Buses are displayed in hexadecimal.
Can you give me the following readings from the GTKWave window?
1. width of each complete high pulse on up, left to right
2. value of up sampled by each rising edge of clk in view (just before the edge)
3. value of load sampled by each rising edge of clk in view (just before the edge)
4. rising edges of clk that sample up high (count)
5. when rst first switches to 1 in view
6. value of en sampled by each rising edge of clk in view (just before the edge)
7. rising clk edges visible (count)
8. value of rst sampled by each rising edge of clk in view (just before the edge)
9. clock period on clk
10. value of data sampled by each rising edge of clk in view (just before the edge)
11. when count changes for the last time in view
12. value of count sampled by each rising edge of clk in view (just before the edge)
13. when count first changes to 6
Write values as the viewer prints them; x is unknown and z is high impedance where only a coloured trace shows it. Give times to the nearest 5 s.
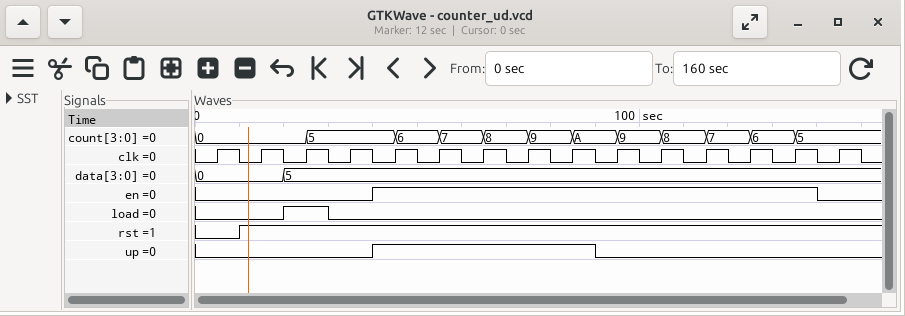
50 s
0 0 0 0 1 1 1 1 1 0 0 0 0 0 0
0 0 1 0 0 0 0 0 0 0 0 0 0 0 0
5
10 s
0 0 0 0 1 1 1 1 1 1 1 1 1 1 0
15
0 1 1 1 1 1 1 1 1 1 1 1 1 1 1
10 s
0, 0, 5, 5, 5, 5, 5, 5, 5, 5, 5, 5, 5, 5, 5
135 s
0, 0, 0, 5, 5, 6, 7, 8, 9, A, 9, 8, 7, 6, 5
45 s
